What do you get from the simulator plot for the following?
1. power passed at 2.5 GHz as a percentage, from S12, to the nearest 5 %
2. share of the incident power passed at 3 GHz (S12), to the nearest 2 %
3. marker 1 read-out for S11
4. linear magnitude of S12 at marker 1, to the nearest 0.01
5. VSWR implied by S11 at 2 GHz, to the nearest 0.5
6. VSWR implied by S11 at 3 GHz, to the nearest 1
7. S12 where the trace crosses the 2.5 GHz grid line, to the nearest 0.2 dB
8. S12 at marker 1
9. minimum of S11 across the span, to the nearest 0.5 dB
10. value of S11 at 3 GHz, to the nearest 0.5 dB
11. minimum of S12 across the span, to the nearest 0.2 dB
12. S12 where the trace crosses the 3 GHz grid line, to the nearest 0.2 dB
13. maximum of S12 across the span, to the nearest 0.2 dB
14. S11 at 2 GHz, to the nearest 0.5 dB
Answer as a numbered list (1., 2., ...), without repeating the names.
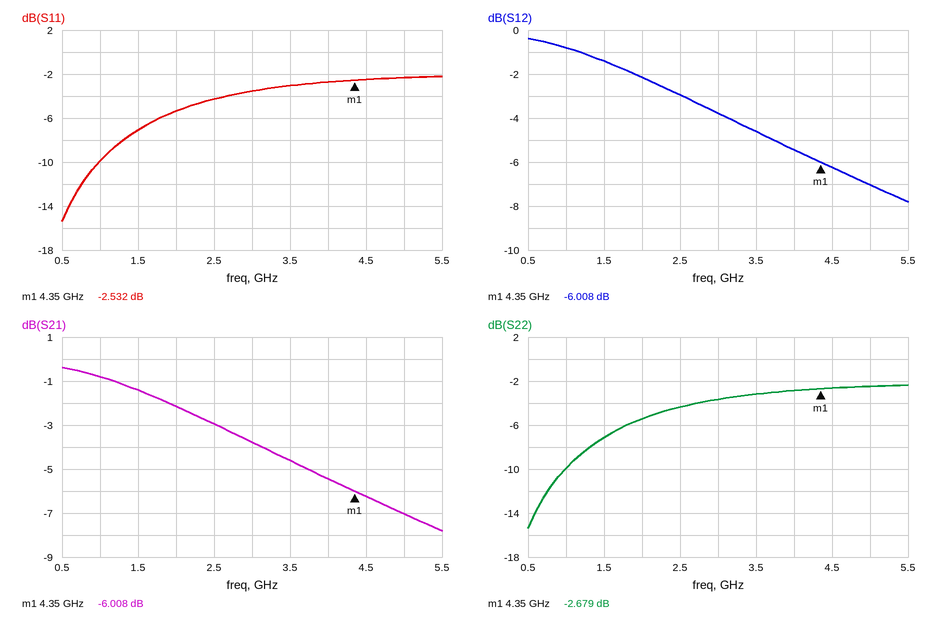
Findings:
1. 50 %
2. 42 %
3. -2.532 dB
4. 0.50
5. 3.5
6. 5
7. -3.0 dB
8. -6.008 dB
9. -15.5 dB
10. -3.5 dB
11. -7.8 dB
12. -3.8 dB
13. -0.4 dB
14. -5.5 dB
